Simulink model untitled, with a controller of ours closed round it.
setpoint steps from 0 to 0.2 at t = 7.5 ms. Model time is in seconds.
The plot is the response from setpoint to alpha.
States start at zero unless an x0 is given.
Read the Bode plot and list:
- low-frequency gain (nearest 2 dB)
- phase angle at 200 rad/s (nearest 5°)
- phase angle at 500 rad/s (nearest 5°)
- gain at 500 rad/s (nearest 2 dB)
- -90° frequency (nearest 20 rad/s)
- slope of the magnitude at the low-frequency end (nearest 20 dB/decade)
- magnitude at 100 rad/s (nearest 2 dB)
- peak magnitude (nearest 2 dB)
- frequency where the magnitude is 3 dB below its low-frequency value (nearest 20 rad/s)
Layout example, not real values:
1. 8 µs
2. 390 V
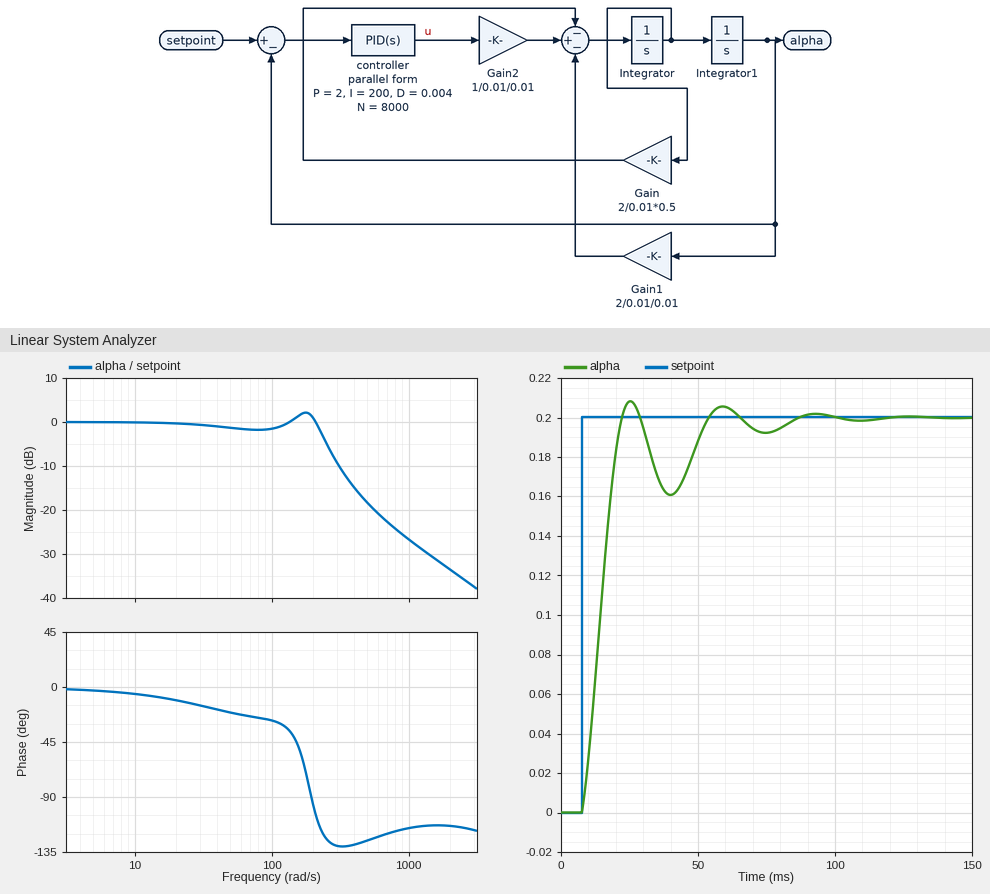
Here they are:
1. 0 dB
2. -95°
3. -125°
4. -18 dB
5. 200 rad/s
6. 0 dB/decade
7. -2 dB
8. 2 dB
9. 240 rad/s
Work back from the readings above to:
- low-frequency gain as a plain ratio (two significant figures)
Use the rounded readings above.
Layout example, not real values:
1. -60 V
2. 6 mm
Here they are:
1. 1.0
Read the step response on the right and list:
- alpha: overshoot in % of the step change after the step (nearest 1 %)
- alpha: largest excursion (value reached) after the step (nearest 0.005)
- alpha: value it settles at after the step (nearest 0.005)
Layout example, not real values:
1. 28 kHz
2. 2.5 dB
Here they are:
1. 4 %
2. 0.210
3. 0.200
